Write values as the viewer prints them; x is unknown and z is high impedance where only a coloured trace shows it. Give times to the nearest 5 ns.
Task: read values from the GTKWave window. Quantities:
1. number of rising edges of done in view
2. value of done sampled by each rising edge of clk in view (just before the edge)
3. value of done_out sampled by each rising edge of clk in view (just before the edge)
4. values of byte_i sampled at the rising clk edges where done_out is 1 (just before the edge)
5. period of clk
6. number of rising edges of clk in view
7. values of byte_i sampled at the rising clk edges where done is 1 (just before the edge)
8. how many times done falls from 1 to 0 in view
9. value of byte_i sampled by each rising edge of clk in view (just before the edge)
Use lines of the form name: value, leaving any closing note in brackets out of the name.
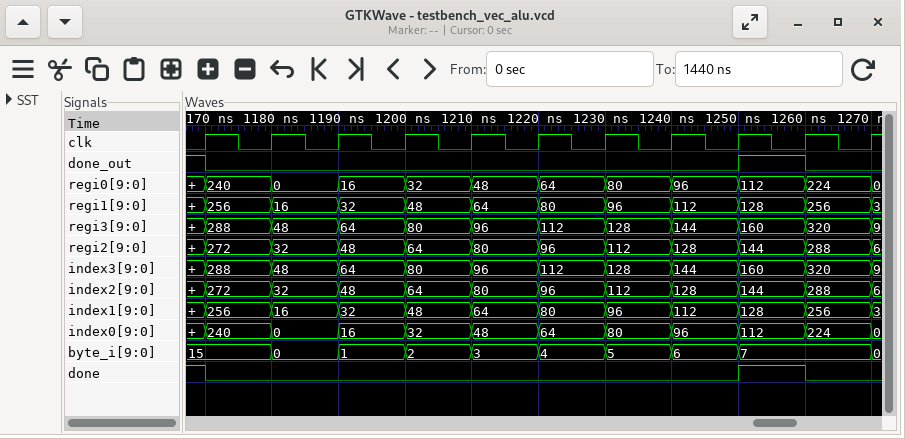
number of rising edges of done in view: 1
value of done sampled by each rising edge of clk in view: 1 0 0 0 0 0 0 0 0 1 0
value of done_out sampled by each rising edge of clk in view: 1 0 0 0 0 0 0 0 0 1 0
values of byte_i sampled at the rising clk edges where done_out is 1: 15, 7
period of clk: 10 ns
number of rising edges of clk in view: 11
values of byte_i sampled at the rising clk edges where done is 1: 15, 7
how many times done falls from 1 to 0 in view: 2
value of byte_i sampled by each rising edge of clk in view: 15, 15, 0, 1, 2, 3, 4, 5, 6, 7, 7
